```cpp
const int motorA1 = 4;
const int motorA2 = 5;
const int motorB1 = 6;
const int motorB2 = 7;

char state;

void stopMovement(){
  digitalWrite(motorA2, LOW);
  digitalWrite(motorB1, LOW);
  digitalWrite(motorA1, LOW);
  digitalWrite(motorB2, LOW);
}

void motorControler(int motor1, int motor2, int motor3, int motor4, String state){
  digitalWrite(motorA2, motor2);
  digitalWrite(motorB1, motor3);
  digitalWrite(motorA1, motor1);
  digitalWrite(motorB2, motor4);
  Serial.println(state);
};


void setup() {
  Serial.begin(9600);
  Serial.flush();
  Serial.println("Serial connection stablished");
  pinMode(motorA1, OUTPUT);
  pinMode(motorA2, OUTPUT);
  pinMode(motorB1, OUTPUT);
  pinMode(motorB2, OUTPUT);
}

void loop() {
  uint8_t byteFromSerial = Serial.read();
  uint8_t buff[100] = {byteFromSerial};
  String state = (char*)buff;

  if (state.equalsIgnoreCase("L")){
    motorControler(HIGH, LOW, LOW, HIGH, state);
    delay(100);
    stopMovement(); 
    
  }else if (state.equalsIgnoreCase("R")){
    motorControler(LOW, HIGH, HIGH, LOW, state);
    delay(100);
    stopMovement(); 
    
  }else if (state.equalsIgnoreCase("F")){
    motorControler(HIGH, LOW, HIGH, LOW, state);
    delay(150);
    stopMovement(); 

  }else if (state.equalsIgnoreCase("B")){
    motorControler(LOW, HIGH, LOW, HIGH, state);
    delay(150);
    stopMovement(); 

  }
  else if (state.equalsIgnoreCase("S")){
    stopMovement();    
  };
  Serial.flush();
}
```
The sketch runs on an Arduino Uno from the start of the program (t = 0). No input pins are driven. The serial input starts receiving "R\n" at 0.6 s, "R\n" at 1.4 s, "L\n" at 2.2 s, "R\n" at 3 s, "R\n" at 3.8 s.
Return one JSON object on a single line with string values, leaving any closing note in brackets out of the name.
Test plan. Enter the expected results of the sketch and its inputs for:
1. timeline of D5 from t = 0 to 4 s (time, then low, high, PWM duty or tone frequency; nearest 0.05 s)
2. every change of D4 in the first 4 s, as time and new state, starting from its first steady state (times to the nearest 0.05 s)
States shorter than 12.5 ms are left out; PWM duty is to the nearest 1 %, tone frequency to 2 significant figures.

{"timeline of D5 from t = 0 to 4 s": "0 s low; 0.6 s high; 0.7 s low; 1.4 s high; 1.5 s low; 3 s high; 3.1 s low; 3.8 s high; 3.9 s low", "every change of D4 in the first 4 s, as time and new state, starting from its first steady state": "0 s low; 2.2 s high; 2.3 s low"}
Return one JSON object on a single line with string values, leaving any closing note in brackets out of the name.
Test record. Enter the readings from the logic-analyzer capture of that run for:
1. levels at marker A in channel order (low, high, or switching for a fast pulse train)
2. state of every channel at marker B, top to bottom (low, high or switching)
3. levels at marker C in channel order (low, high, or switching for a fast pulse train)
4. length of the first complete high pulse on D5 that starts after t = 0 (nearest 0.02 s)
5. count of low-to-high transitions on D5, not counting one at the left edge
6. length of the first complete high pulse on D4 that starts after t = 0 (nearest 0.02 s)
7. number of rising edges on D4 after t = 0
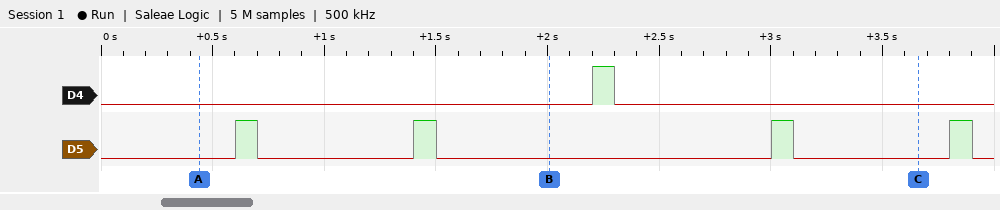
{"levels at marker A in channel order": "D4 low, D5 low", "state of every channel at marker B, top to bottom": "D4 low, D5 low", "levels at marker C in channel order": "D4 low, D5 low", "length of the first complete high pulse on D5 that starts after t = 0": "0.10 s", "count of low-to-high transitions on D5, not counting one at the left edge": "4", "length of the first complete high pulse on D4 that starts after t = 0": "0.10 s", "number of rising edges on D4 after t = 0": "1"}
